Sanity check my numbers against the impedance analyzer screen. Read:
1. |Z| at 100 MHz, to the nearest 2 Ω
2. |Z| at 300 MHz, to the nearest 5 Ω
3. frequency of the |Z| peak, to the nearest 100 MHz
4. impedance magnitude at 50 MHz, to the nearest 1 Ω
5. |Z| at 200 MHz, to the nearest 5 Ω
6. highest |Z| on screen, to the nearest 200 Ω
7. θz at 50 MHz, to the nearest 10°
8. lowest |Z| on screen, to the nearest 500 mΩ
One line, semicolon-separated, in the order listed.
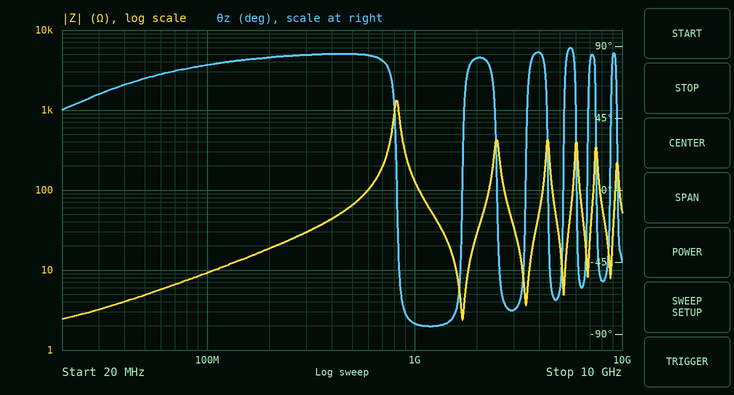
10 Ω; 30 Ω; 800 MHz; 5 Ω; 20 Ω; 1.4 kΩ; 70°; 2.5 Ω
